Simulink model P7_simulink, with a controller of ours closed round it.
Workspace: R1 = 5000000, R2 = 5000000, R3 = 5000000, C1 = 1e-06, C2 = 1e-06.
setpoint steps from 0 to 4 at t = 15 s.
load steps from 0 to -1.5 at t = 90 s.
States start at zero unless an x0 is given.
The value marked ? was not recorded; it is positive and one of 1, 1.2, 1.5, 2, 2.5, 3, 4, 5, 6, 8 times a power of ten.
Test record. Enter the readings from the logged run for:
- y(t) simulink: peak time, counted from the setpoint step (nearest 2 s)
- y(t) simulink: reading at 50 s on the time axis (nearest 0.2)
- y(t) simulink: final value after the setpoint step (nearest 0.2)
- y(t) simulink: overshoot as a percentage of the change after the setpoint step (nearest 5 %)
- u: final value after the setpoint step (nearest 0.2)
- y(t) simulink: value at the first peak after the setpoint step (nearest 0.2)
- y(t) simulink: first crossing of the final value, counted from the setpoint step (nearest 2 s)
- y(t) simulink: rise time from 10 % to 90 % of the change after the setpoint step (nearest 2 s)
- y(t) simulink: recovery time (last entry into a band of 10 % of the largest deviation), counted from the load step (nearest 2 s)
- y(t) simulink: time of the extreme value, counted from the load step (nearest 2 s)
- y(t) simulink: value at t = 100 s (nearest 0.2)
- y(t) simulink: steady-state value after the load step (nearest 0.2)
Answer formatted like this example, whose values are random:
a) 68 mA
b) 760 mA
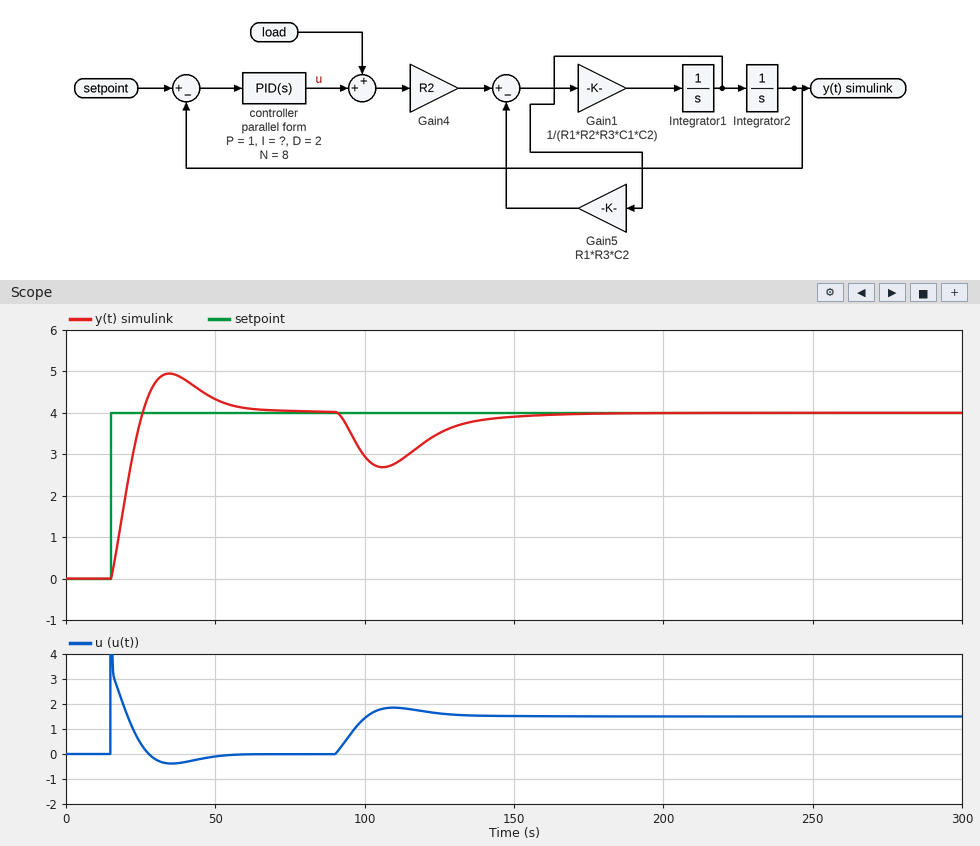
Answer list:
a) 20 s
b) 4.4
c) 4.0
d) 25 %
e) 0.0
f) 5.0
g) 10 s
h) 8 s
i) 54 s
j) 16 s
k) 3.0
l) 4.0
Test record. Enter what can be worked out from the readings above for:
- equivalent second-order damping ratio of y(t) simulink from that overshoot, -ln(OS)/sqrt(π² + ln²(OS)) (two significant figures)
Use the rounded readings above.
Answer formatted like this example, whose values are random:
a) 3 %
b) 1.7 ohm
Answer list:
a) 0.40
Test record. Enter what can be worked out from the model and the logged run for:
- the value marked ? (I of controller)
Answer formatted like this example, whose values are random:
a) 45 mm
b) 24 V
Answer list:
a) 0.04
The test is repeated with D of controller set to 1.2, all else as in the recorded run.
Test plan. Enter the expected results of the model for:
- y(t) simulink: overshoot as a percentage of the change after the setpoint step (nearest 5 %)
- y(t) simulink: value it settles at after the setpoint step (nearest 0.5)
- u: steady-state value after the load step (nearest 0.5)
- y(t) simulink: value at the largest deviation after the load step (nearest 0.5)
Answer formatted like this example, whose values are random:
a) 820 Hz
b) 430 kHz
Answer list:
a) 30 %
b) 4.0
c) 1.5
d) 2.5
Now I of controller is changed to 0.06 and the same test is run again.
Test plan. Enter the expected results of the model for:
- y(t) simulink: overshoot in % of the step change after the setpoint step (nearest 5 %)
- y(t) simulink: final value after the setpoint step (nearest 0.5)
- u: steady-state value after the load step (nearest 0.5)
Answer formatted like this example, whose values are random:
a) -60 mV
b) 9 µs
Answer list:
a) 30 %
b) 4.0
c) 1.5
